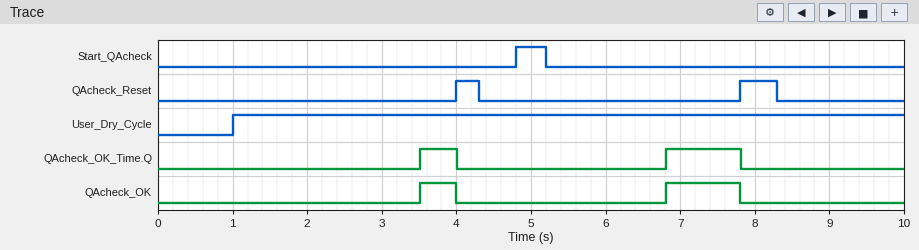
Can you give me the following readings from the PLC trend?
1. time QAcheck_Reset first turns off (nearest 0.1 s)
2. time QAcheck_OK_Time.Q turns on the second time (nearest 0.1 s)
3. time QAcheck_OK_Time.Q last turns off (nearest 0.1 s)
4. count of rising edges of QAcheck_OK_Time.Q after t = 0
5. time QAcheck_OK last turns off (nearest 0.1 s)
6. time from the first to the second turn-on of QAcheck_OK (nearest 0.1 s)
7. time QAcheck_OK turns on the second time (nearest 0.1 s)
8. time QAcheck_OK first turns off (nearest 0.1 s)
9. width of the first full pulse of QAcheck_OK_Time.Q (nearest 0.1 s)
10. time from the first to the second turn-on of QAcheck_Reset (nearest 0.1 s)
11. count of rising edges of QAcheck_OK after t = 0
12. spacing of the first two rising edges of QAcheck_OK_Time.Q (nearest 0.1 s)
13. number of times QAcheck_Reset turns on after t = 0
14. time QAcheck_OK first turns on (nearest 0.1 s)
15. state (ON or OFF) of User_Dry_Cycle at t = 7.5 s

4.3 s
6.8 s
7.8 s
2
7.8 s
3.3 s
6.8 s
4.0 s
0.5 s
3.8 s
2
3.3 s
2
3.5 s
ON
